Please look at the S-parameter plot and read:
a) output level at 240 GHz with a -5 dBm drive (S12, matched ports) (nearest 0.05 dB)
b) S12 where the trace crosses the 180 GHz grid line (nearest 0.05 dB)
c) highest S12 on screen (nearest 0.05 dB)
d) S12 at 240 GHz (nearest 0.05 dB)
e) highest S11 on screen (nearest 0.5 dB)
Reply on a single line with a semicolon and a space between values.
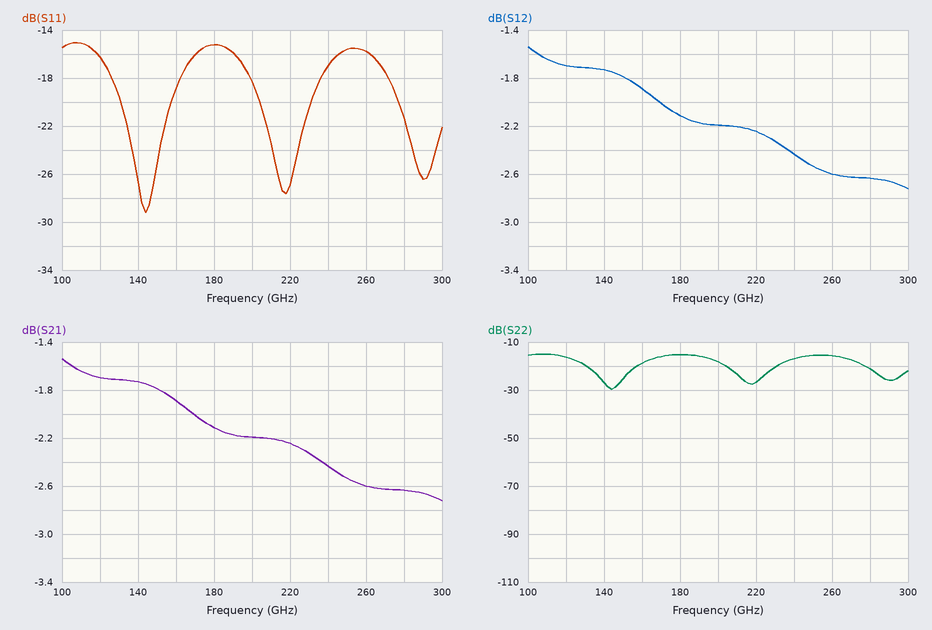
-7.45 dBm; -2.10 dB; -1.55 dB; -2.45 dB; -15.0 dB
